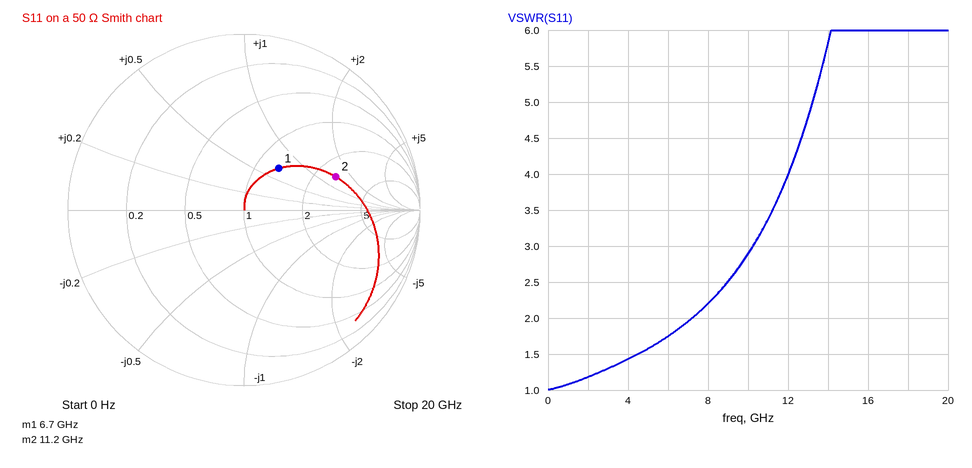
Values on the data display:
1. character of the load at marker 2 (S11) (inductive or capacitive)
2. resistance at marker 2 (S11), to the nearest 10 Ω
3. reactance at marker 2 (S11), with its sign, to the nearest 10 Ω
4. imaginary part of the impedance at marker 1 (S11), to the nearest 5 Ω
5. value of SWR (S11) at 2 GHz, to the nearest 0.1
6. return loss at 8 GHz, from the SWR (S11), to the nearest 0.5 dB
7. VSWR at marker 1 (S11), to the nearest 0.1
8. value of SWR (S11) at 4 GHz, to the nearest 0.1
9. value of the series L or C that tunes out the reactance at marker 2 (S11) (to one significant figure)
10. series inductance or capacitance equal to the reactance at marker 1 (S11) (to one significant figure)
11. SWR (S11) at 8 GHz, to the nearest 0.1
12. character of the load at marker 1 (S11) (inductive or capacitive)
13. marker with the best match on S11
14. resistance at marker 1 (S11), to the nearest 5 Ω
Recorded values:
inductive
130 Ω
+70 Ω
+35 Ω
1.2
8.5 dB
1.9
1.4
200 fF
800 pH
2.2
inductive
marker 1
65 Ω
